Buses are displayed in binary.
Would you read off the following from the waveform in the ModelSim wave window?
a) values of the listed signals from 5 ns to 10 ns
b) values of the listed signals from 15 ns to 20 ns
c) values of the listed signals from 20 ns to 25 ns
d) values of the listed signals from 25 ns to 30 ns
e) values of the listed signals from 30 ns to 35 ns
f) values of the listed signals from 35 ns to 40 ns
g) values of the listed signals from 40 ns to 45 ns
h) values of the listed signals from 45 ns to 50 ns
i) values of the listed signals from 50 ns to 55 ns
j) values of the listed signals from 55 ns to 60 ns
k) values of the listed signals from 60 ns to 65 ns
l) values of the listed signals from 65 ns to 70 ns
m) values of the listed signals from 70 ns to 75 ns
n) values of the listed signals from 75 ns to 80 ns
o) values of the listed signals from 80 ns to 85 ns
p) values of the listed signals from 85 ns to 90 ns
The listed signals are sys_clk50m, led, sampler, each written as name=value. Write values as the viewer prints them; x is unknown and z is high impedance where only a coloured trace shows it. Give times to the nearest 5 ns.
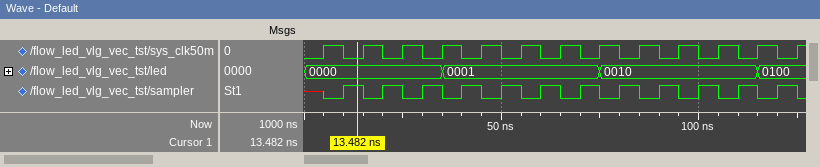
sys_clk50m=1, led=0000, sampler=0
sys_clk50m=1, led=0000, sampler=0
sys_clk50m=0, led=0000, sampler=1
sys_clk50m=1, led=0000, sampler=0
sys_clk50m=0, led=0000, sampler=1
sys_clk50m=1, led=0001, sampler=0
sys_clk50m=0, led=0001, sampler=1
sys_clk50m=1, led=0001, sampler=0
sys_clk50m=0, led=0001, sampler=1
sys_clk50m=1, led=0001, sampler=0
sys_clk50m=0, led=0001, sampler=1
sys_clk50m=1, led=0001, sampler=0
sys_clk50m=0, led=0001, sampler=1
sys_clk50m=1, led=0010, sampler=0
sys_clk50m=0, led=0010, sampler=1
sys_clk50m=1, led=0010, sampler=0
